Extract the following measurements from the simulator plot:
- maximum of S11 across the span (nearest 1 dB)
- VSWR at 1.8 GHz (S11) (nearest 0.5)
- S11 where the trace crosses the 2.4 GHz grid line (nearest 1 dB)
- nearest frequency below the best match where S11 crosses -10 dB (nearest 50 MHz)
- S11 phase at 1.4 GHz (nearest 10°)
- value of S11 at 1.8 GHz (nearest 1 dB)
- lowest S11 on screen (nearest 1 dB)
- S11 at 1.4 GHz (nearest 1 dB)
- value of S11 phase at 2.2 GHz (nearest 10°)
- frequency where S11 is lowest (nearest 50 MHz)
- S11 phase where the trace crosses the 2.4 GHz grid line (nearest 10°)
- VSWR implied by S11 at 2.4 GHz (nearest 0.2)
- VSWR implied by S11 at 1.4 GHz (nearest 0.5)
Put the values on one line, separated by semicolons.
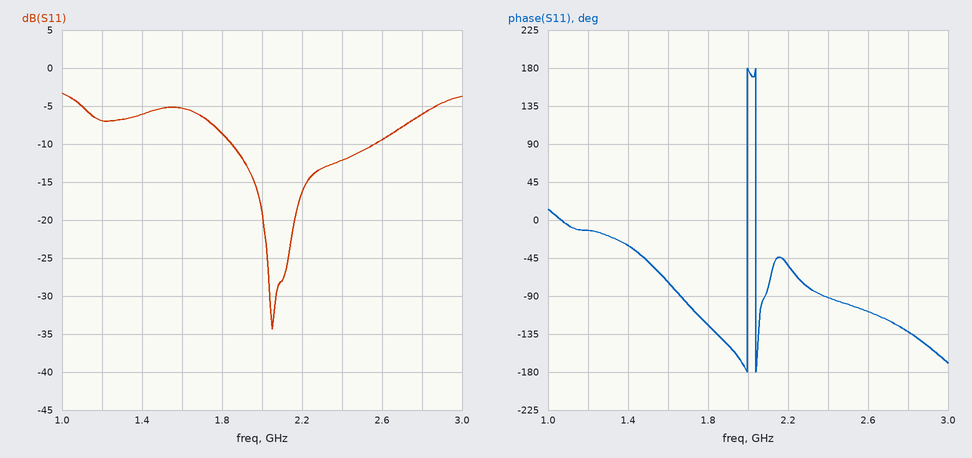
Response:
-3 dB; 2.0; -12 dB; 1.85 GHz; -30°; -9 dB; -34 dB; -6 dB; -50°; 2.05 GHz; -90°; 1.6; 3.0
